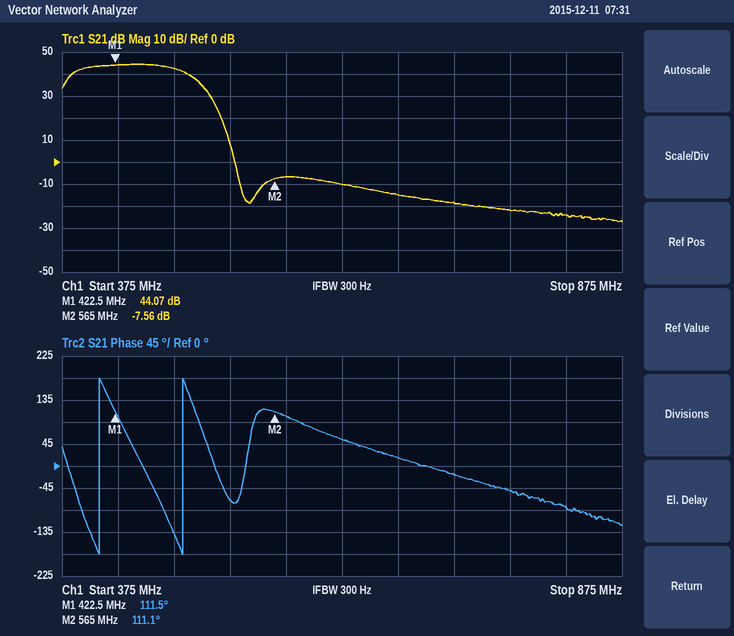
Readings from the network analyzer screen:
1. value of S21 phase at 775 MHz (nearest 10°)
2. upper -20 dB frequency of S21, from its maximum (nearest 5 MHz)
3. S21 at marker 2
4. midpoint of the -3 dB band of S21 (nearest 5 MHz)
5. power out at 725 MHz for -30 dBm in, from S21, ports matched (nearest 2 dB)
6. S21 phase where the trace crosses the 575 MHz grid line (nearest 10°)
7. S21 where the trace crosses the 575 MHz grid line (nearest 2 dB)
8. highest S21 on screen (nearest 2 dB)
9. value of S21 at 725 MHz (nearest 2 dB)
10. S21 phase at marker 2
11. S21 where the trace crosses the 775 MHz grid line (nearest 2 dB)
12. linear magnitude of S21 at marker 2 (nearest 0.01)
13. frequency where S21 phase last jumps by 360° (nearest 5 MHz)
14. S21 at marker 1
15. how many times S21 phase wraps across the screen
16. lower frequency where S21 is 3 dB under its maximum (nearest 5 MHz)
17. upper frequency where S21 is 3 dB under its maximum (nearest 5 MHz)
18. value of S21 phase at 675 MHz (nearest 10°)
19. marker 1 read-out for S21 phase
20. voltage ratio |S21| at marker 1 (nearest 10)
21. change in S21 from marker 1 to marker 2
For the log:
-50°
515 MHz
-7.56 dB
435 MHz
-48 dBm
100°
-6 dB
44 dB
-18 dB
111.1°
-22 dB
0.42
485 MHz
44.07 dB
2
390 MHz
480 MHz
20°
111.5°
160
-51.63 dB
